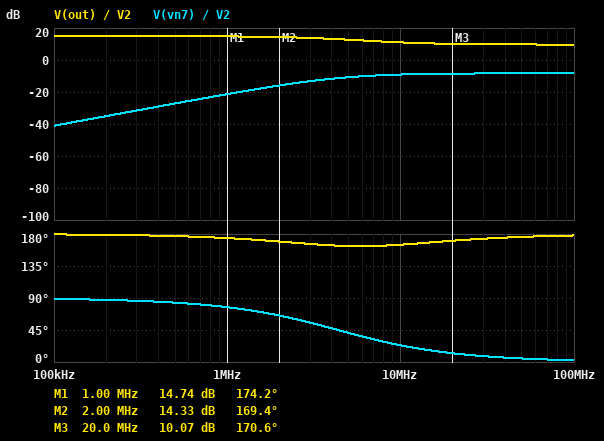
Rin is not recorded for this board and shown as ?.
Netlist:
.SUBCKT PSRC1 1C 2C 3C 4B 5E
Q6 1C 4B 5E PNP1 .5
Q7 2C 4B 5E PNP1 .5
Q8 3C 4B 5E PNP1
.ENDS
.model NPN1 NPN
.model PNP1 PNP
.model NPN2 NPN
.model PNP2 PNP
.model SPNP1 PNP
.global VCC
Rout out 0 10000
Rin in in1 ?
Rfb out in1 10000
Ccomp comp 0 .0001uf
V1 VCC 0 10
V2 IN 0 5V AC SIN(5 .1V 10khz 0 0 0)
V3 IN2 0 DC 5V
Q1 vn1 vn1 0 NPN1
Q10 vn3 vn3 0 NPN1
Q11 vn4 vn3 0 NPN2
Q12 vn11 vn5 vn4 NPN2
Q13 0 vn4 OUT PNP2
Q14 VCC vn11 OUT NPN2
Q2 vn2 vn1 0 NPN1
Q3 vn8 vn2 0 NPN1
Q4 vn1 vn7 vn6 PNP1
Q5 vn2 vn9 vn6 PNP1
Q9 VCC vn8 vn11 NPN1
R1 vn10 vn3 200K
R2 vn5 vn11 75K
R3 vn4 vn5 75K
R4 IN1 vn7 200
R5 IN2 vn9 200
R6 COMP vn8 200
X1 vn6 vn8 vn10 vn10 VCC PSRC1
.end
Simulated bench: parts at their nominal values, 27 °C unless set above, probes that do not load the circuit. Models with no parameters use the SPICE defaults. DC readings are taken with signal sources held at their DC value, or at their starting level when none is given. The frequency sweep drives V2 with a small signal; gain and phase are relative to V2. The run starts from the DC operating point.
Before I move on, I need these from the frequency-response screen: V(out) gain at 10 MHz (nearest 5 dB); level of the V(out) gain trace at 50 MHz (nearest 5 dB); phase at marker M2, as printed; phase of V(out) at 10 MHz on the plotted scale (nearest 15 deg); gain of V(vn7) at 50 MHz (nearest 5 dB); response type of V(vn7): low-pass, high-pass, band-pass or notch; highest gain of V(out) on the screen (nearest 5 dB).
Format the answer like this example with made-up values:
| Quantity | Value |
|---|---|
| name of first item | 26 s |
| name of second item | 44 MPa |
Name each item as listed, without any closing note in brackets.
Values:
| Quantity | Value |
|---|---|
| V(out) gain at 10 MHz | 10 dB |
| level of the V(out) gain trace at 50 MHz | 10 dB |
| phase at marker M2, as printed | 169.4 deg |
| phase of V(out) at 10 MHz on the plotted scale | 165 deg |
| gain of V(vn7) at 50 MHz | -10 dB |
| response type of V(vn7): low-pass, high-pass, band-pass or notch | high-pass |
| highest gain of V(out) on the screen | 15 dB |
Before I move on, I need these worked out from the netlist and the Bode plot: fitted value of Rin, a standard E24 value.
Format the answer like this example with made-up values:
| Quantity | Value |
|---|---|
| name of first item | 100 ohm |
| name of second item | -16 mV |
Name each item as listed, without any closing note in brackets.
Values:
| Quantity | Value |
|---|---|
| fitted value of Rin, a standard E24 value | 1.8 kΩ |
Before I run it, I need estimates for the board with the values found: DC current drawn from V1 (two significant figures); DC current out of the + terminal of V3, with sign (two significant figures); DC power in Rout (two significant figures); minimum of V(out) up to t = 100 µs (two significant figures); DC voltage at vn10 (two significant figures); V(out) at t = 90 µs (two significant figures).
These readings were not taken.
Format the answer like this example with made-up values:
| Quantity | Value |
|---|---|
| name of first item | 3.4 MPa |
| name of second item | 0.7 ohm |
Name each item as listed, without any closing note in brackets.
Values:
| Quantity | Value |
|---|---|
| DC current drawn from V1 | 630 µA |
| DC current out of the + terminal of V3, with sign | -100 nA |
| DC power in Rout | 2.5 mW |
| minimum of V(out) up to t = 100 µs | 4.4 V |
| DC voltage at vn10 | 9.3 V |
| V(out) at t = 90 µs | 5.3 V |
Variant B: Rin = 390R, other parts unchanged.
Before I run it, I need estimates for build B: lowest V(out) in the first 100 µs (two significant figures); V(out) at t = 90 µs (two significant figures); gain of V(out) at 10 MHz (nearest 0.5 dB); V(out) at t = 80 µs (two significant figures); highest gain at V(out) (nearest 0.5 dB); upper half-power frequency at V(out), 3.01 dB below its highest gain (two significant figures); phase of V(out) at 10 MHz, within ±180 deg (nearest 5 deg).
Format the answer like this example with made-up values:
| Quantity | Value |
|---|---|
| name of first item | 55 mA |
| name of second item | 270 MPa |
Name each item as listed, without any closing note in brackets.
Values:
| Quantity | Value |
|---|---|
| lowest V(out) in the first 100 µs | 2.4 V |
| V(out) at t = 90 µs | 6.5 V |
| gain of V(out) at 10 MHz | 17.5 dB |
| V(out) at t = 80 µs | 7.4 V |
| highest gain at V(out) | 28.0 dB |
| upper half-power frequency at V(out), 3.01 dB below its highest gain | 1.9 MHz |
| phase of V(out) at 10 MHz, within ±180 deg | 150 deg |
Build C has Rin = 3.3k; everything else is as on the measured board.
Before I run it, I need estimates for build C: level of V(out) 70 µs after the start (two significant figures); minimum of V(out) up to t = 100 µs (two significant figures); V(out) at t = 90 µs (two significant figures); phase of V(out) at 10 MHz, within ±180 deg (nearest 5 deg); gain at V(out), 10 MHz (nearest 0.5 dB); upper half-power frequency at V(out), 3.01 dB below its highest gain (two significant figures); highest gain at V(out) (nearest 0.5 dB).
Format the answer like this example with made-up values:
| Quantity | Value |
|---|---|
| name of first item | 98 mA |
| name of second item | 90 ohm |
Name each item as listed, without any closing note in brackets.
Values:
| Quantity | Value |
|---|---|
| level of V(out) 70 µs after the start | 5.3 V |
| minimum of V(out) up to t = 100 µs | 4.7 V |
| V(out) at t = 90 µs | 5.2 V |
| phase of V(out) at 10 MHz, within ±180 deg | 170 deg |
| gain at V(out), 10 MHz | 7.0 dB |
| upper half-power frequency at V(out), 3.01 dB below its highest gain | 15 MHz |
| highest gain at V(out) | 9.5 dB |
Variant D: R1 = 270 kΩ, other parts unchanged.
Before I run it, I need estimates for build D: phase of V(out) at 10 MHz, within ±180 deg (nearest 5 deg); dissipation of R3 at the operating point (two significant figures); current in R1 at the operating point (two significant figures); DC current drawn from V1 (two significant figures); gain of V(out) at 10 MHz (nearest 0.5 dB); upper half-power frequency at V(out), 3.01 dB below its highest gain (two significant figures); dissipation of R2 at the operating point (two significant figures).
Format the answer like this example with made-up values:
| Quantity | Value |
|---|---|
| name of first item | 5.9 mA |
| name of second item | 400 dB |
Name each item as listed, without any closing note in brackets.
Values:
| Quantity | Value |
|---|---|
| phase of V(out) at 10 MHz, within ±180 deg | 160 deg |
| dissipation of R3 at the operating point | 6.1 µW |
| current in R1 at the operating point | 32 µA |
| DC current drawn from V1 | 600 µA |
| gain of V(out) at 10 MHz | 10.0 dB |
| upper half-power frequency at V(out), 3.01 dB below its highest gain | 5.0 MHz |
| dissipation of R2 at the operating point | 6.4 µW |
